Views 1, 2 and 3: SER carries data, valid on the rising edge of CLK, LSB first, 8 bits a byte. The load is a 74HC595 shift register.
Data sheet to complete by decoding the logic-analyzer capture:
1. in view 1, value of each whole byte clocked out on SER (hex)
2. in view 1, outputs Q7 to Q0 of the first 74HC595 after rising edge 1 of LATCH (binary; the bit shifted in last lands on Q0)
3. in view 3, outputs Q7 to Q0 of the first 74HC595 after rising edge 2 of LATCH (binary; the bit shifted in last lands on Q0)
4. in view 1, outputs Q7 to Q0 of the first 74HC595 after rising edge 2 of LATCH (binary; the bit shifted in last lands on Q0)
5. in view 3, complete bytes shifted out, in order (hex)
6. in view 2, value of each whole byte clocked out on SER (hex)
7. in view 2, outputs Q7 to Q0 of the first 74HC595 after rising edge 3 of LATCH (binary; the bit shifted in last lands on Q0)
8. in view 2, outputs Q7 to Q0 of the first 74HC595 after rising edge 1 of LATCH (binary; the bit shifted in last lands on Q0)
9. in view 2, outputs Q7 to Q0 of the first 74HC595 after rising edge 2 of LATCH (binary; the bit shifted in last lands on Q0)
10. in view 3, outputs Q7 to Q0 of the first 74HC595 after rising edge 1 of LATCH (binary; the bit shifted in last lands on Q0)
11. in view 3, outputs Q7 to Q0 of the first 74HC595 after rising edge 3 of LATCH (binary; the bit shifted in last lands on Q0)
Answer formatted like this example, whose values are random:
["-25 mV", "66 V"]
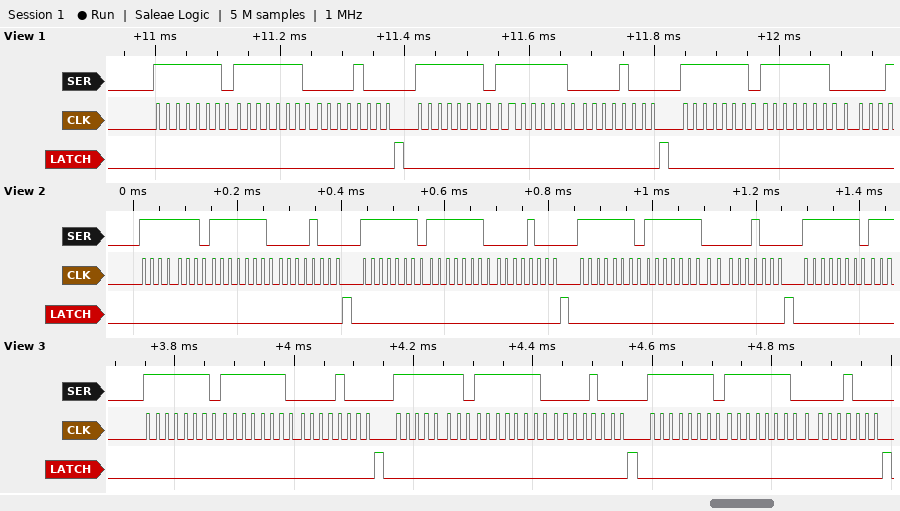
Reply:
["0x7F 0x7F 0x10 0x7F 0x7F 0x10 0x7F 0x7F", "00001000", "00001000", "00001000", "7F 7F 10 7F 7F 10 7F 7F 10", "7F 7F 10 7F 7F 10 7F 7F 10 7F", "00001000", "00001000", "00001000", "00001000", "00001000"]
